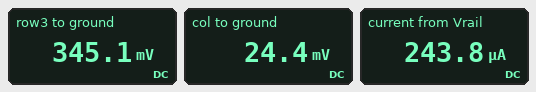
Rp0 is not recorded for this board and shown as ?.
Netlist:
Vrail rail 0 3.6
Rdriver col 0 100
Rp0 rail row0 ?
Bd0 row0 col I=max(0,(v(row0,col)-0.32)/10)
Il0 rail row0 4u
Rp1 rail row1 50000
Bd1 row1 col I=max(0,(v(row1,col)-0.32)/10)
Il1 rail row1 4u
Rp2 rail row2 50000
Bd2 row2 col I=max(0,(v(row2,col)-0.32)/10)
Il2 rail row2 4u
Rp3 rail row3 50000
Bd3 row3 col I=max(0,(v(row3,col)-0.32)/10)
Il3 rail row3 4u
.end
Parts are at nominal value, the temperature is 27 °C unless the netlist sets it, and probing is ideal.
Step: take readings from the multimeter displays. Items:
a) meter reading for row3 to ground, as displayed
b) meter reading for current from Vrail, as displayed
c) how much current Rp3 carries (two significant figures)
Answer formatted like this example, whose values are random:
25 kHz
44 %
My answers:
345.1 mV
243.8 µA
65 µA
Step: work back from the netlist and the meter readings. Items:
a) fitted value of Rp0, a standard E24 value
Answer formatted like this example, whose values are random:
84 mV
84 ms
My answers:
100 kΩ
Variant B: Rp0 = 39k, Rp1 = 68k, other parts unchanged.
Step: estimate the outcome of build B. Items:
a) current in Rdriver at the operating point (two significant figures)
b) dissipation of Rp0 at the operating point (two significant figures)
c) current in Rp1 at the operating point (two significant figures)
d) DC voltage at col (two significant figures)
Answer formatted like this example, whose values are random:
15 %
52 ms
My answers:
280 µA
270 µW
48 µA
28 mV
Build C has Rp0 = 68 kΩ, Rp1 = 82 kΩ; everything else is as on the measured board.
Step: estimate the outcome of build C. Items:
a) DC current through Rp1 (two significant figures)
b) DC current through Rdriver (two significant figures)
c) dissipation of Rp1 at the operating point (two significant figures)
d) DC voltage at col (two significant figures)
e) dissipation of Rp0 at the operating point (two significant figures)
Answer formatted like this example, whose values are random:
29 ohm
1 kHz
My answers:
40 µA
230 µA
130 µW
23 mV
160 µW
